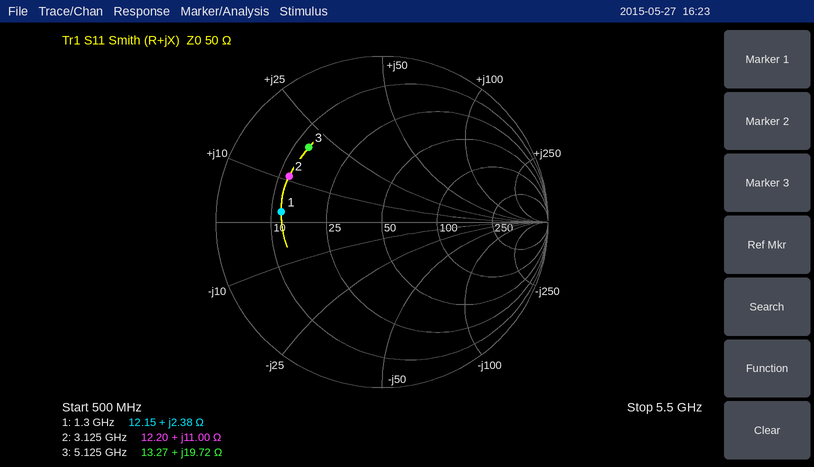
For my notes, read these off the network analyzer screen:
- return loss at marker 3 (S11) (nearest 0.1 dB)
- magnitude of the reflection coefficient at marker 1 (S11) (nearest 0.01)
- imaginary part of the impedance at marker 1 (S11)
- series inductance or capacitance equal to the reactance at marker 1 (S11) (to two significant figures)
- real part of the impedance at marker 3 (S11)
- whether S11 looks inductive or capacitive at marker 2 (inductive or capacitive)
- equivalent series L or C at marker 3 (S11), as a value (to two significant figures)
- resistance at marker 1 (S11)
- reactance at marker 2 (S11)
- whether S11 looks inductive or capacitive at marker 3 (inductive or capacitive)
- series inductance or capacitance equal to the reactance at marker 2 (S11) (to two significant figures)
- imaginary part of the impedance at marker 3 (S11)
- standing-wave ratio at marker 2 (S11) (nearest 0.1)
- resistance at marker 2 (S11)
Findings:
4.0 dB
0.61
+2.38 Ω
290 pH
13.27 Ω
inductive
610 pH
12.15 Ω
+11.00 Ω
inductive
560 pH
+19.72 Ω
4.3
12.20 Ω
